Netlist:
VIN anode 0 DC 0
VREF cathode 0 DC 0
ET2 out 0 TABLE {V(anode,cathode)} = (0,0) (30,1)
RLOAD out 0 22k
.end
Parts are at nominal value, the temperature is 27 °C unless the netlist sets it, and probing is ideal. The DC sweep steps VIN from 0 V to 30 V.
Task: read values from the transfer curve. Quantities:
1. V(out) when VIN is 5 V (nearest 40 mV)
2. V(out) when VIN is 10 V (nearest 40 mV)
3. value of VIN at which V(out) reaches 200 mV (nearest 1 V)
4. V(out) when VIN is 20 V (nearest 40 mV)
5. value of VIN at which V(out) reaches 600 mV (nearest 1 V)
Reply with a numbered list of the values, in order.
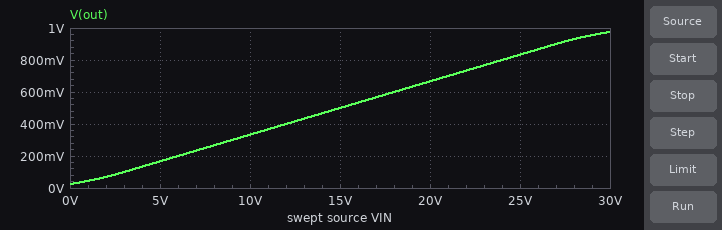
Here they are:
1. 160 mV
2. 320 mV
3. 6 V
4. 680 mV
5. 18 V
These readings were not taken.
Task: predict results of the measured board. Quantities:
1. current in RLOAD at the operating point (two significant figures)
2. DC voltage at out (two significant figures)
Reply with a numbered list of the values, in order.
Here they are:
1. 1.1 µA
2. 25 mV
